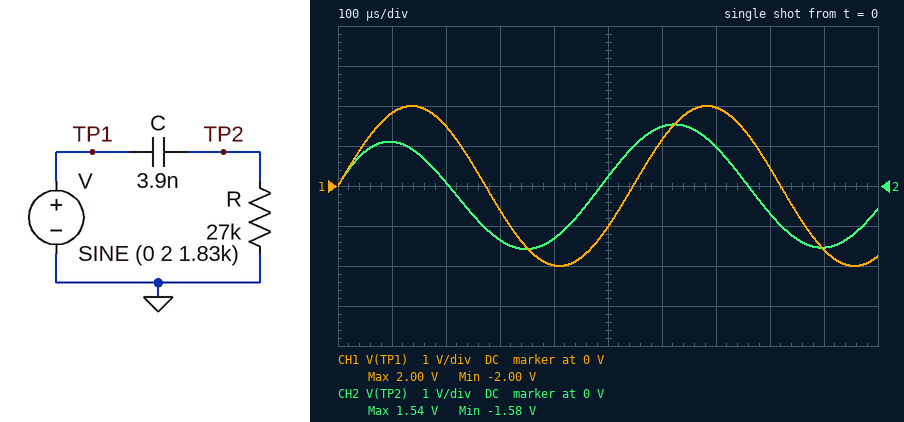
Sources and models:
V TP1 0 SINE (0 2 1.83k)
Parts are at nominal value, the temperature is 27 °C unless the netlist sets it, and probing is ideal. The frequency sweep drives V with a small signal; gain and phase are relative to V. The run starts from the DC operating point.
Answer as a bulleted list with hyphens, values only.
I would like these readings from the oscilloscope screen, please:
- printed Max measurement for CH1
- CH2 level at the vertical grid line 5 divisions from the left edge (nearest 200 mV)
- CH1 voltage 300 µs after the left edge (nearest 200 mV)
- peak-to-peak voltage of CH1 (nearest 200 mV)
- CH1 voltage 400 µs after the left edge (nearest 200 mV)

- 2.00 V
- 200 mV
- -600 mV
- 4.0 V
- -2.0 V
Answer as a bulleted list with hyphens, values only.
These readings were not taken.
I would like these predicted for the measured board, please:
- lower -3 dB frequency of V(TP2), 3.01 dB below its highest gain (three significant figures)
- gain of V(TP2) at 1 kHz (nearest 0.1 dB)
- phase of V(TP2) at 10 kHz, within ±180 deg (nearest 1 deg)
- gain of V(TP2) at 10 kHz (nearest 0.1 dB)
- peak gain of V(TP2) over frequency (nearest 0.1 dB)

- 1.51 kHz
- -5.2 dB
- 9 deg
- -0.1 dB
- 0 dB
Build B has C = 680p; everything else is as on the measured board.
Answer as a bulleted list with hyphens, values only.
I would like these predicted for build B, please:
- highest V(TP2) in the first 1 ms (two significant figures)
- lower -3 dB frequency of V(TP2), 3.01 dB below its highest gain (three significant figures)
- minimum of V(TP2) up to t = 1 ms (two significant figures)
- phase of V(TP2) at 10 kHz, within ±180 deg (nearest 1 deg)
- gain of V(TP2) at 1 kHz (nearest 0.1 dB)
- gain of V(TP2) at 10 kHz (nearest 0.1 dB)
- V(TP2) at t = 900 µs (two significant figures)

- 410 mV
- 8.67 kHz
- -410 mV
- 41 deg
- -18.8 dB
- -2.4 dB
- -310 mV
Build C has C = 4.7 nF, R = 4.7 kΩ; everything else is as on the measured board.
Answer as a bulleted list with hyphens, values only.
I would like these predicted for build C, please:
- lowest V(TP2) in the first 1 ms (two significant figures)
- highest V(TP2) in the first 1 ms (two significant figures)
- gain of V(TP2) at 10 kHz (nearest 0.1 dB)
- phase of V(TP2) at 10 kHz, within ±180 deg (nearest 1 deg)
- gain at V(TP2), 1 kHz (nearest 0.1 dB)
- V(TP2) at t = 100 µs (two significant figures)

- -490 mV
- 490 mV
- -1.8 dB
- 36 deg
- -17.2 dB
- 300 mV
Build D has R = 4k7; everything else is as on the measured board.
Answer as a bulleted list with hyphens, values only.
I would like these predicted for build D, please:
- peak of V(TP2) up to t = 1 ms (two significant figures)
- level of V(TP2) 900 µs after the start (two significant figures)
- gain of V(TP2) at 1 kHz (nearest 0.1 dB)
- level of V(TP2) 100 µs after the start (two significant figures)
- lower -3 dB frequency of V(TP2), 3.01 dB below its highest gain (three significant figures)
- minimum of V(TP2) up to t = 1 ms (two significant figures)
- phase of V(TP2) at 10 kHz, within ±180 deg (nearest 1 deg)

- 410 mV
- -310 mV
- -18.8 dB
- 240 mV
- 8.68 kHz
- -410 mV
- 41 deg
